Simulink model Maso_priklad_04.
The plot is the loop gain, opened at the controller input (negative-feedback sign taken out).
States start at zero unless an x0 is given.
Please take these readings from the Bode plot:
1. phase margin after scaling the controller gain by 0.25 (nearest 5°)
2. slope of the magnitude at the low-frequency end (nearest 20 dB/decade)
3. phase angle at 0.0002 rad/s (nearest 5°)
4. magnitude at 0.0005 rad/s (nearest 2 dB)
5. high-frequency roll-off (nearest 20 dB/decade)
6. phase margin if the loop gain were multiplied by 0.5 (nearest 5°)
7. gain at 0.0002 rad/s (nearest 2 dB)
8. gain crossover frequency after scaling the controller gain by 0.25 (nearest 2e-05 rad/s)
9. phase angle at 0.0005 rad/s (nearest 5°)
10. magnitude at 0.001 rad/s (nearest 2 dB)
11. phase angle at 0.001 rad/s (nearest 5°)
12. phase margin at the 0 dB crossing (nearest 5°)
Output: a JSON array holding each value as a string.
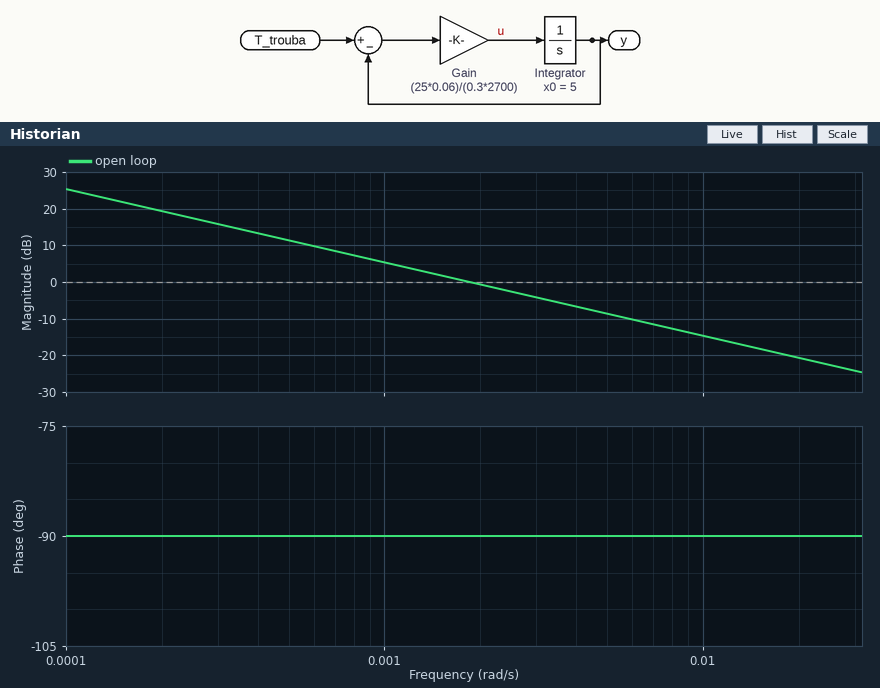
["90°", "-20 dB/decade", "-90°", "12 dB", "-20 dB/decade", "90°", "20 dB", "0.00046 rad/s", "-90°", "6 dB", "-90°", "90°"]
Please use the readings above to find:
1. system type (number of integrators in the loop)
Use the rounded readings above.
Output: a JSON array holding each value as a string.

["1"]
